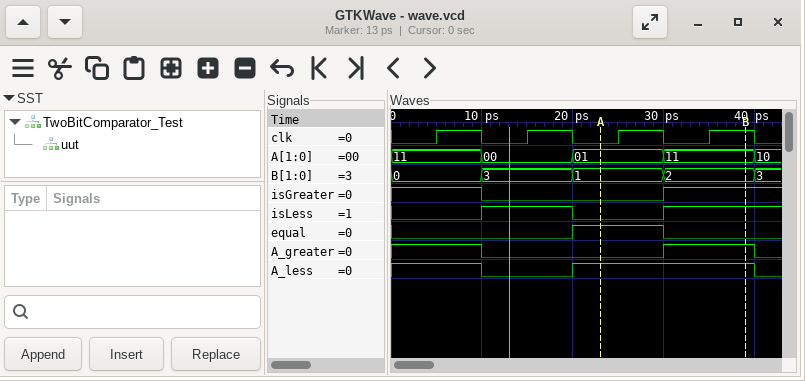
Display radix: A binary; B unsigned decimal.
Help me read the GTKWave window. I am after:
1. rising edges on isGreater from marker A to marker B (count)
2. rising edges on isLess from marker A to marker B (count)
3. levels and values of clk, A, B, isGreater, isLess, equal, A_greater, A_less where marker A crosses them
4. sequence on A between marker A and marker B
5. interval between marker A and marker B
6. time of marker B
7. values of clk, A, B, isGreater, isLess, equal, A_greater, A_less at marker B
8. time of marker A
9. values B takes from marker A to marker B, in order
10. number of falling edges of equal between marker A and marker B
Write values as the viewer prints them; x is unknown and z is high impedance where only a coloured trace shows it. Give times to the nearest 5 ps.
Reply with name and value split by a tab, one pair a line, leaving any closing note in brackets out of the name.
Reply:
rising edges on isGreater from marker A to marker B	1
rising edges on isLess from marker A to marker B	1
levels and values of clk, A, B, isGreater, isLess, equal, A_greater, A_less where marker A crosses them	clk=0, A=01, B=1, isGreater=0, isLess=0, equal=1, A_greater=0, A_less=1
sequence on A between marker A and marker B	01, 11
interval between marker A and marker B	15 ps
time of marker B	40 ps
values of clk, A, B, isGreater, isLess, equal, A_greater, A_less at marker B	clk=1, A=11, B=2, isGreater=1, isLess=1, equal=0, A_greater=1, A_less=1
time of marker A	25 ps
values B takes from marker A to marker B, in order	1, 2
number of falling edges of equal between marker A and marker B	1
